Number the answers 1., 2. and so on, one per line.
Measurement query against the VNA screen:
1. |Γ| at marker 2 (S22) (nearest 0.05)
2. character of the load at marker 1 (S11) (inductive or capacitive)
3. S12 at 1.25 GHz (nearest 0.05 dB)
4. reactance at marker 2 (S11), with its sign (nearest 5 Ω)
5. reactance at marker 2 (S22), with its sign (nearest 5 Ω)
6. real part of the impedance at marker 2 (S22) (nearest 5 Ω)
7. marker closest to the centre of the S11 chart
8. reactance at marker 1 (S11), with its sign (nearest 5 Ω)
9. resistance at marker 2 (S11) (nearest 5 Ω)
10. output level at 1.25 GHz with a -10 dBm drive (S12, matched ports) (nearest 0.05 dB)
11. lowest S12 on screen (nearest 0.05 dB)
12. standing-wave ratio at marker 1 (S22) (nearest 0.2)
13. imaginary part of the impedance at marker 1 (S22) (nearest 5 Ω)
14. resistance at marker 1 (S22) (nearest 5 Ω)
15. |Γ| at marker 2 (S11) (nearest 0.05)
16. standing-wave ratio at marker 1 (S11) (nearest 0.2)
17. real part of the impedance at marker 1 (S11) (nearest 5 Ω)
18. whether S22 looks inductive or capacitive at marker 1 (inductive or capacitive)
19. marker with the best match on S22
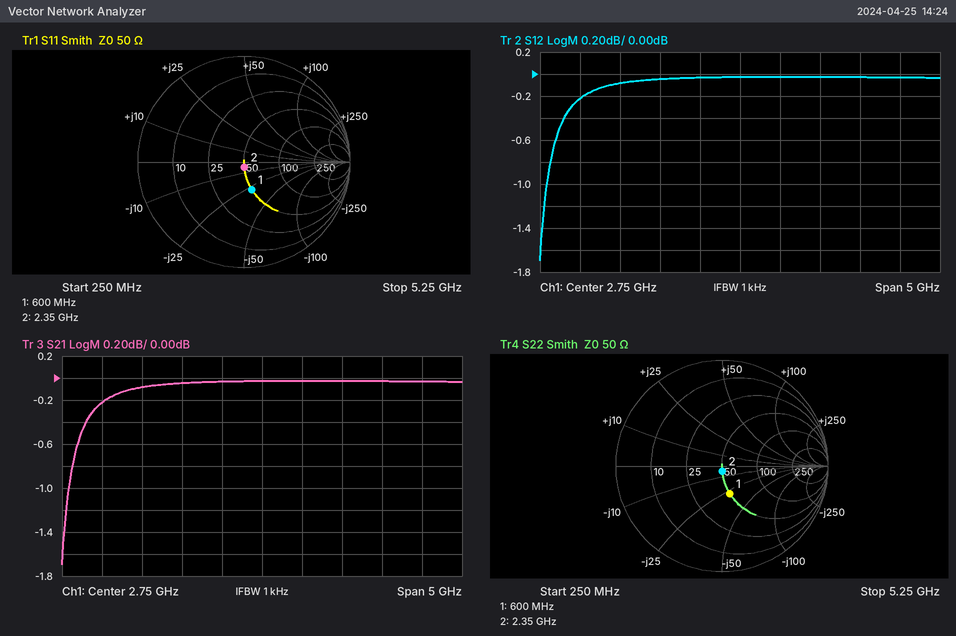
1. 0.05
2. capacitive
3. -0.10 dB
4. -5 Ω
5. -5 Ω
6. 50 Ω
7. marker 2
8. -30 Ω
9. 50 Ω
10. -10.10 dBm
11. -1.70 dB
12. 1.8
13. -30 Ω
14. 50 Ω
15. 0.05
16. 1.8
17. 50 Ω
18. capacitive
19. marker 2
